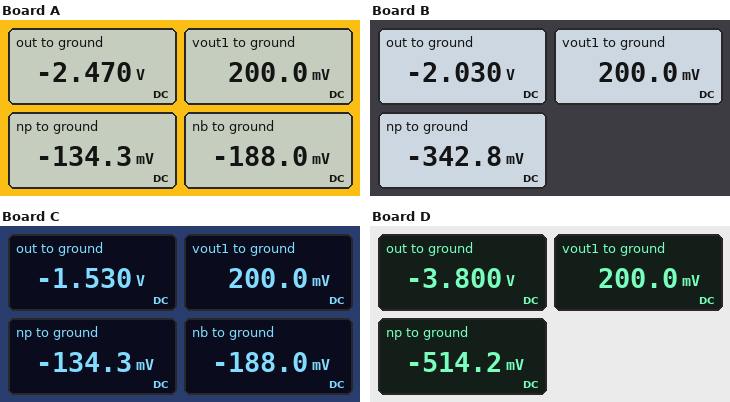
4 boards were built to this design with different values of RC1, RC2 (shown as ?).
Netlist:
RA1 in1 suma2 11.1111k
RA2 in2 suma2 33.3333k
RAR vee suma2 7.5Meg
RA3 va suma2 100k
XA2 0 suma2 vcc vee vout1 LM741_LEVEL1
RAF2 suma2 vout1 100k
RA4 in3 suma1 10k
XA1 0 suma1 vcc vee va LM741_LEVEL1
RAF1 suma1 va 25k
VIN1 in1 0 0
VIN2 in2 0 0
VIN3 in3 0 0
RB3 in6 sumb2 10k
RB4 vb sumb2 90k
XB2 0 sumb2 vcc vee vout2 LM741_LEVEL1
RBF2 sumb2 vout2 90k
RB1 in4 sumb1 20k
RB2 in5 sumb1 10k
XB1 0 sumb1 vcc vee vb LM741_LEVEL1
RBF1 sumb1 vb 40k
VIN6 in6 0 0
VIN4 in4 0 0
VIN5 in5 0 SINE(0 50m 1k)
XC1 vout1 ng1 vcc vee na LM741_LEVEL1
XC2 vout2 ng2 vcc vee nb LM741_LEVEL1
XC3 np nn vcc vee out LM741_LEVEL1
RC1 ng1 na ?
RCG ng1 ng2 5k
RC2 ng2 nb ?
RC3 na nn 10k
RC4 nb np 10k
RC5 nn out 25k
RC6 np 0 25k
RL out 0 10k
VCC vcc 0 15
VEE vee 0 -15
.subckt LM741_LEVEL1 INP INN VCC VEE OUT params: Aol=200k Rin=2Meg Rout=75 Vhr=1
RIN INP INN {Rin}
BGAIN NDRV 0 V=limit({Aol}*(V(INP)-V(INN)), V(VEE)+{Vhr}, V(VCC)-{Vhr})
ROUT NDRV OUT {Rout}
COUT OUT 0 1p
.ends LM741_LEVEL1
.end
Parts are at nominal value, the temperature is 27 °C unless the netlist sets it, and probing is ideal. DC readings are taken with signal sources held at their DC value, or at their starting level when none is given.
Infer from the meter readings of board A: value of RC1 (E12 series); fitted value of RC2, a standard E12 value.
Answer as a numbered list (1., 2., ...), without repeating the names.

1. 15 kΩ
2. 4.7 kΩ
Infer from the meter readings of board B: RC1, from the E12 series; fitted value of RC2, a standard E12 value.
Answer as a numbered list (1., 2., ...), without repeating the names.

1. 3.3 kΩ
2. 12 kΩ
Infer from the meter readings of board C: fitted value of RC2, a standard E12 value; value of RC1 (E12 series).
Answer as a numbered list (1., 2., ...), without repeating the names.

1. 4.7 kΩ
2. 5.6 kΩ
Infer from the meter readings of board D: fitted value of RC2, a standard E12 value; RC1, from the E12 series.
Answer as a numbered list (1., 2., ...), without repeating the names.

1. 18 kΩ
2. 15 kΩ
